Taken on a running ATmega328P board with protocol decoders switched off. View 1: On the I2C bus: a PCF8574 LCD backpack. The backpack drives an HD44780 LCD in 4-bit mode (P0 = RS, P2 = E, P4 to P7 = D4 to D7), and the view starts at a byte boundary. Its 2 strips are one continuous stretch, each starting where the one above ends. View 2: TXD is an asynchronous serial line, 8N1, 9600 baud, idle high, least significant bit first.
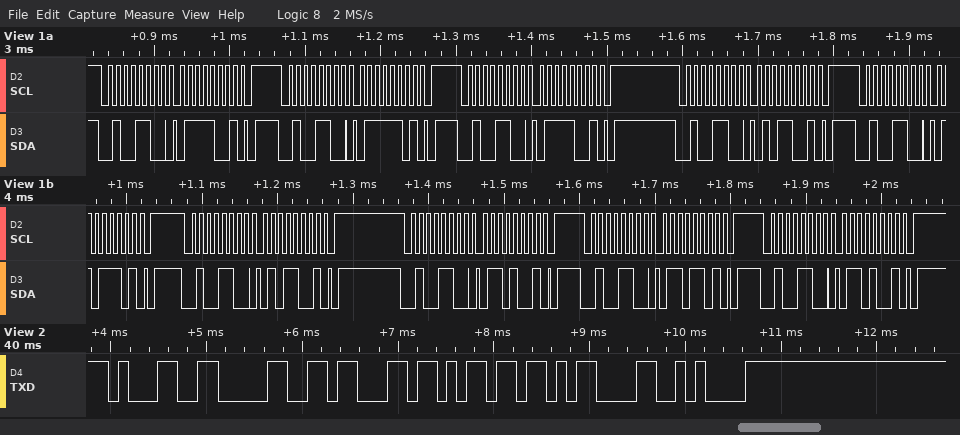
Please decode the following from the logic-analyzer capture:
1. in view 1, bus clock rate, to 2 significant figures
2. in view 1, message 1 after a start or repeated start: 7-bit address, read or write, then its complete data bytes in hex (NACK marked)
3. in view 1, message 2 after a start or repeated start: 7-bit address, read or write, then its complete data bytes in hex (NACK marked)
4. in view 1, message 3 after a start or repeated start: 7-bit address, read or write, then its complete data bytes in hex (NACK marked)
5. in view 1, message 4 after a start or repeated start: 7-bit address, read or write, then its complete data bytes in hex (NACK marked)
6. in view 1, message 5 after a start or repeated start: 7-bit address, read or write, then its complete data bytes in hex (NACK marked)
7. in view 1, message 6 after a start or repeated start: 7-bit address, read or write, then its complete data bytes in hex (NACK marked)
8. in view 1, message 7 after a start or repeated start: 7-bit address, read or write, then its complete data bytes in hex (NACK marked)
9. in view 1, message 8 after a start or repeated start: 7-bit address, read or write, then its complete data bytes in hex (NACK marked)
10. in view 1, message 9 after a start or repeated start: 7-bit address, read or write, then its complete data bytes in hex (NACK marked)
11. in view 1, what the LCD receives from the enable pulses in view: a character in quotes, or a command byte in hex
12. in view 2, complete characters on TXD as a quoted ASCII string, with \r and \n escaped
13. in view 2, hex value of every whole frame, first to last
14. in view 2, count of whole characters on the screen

100 kHz
0x26 write: 79
0x26 write: 7D
0x26 write: 79
0x26 write: 59
0x26 write: 5D
0x26 write: 59
0x26 write: 69
0x26 write: 6D
0x26 write: 69
'u'
"10cm\r\n"
31 30 63 6D 0D 0A
6
